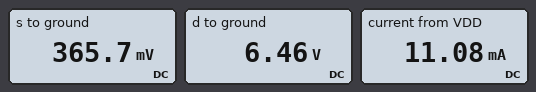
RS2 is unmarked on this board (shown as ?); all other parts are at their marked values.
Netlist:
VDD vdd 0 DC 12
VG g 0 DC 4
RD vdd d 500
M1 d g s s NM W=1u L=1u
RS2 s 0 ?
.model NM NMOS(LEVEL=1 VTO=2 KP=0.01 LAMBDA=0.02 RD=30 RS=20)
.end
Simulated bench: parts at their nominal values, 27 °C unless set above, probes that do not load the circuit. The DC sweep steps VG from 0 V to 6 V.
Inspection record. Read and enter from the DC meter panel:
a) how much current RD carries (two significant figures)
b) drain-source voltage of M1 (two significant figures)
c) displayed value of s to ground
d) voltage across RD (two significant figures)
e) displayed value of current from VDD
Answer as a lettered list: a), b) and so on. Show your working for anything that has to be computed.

a) (12 V - 6.46 V) / 500 Ω = 11 mA
b) 6.46 V - 365.7 mV = 6.1 V
c) 365.7 mV
d) 12 V - 6.46 V = 5.5 V
e) 11.08 mA
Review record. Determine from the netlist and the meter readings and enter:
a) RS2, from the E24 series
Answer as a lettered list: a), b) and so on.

a) 33 Ω
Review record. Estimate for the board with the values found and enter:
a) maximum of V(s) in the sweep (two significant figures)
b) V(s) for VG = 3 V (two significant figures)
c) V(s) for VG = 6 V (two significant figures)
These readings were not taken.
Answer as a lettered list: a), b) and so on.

a) 640 mV
b) 130 mV
c) 640 mV
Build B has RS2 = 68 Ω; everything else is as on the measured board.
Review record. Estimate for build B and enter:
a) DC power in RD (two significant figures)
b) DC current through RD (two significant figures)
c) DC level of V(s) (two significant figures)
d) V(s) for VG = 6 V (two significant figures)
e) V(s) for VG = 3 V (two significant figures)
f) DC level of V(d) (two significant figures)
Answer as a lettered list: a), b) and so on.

a) 38 mW
b) 8.7 mA
c) 590 mV
d) 1.2 V
e) 210 mV
f) 7.7 V
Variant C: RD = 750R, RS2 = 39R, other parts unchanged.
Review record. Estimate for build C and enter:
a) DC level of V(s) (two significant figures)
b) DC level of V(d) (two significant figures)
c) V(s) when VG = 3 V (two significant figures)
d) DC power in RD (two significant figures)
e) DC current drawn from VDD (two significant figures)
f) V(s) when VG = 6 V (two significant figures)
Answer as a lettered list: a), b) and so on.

a) 400 mV
b) 4.3 V
c) 140 mV
d) 80 mW
e) 10 mA
f) 540 mV
